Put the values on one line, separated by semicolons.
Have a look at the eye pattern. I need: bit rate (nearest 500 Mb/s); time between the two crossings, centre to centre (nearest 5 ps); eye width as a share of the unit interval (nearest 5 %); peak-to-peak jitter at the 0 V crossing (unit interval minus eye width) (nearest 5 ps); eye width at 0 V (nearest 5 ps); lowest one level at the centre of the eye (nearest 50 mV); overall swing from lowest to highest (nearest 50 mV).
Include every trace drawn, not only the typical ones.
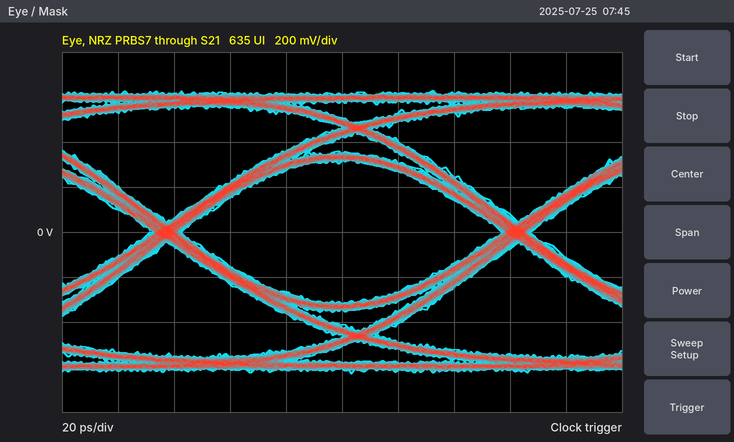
8.0 Gb/s; 125 ps; 90 %; 10 ps; 115 ps; 300 mV; 1.25 V
